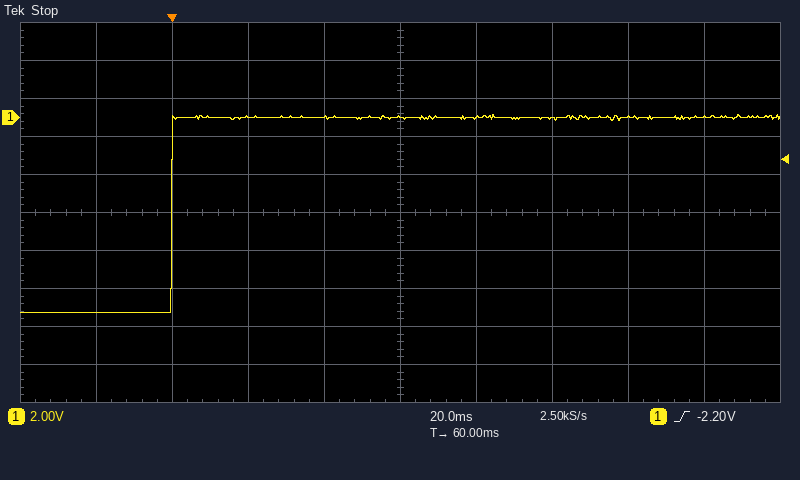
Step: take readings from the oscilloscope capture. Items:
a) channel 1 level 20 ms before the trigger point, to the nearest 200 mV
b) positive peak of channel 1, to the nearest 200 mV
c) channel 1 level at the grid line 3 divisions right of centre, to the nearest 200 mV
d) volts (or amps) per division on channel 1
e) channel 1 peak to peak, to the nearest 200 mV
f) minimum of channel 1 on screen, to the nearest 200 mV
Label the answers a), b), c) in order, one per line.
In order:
a) -10.2 V
b) 200 mV
c) 0.0 V
d) 2 V
e) 10.4 V
f) -10.2 V
